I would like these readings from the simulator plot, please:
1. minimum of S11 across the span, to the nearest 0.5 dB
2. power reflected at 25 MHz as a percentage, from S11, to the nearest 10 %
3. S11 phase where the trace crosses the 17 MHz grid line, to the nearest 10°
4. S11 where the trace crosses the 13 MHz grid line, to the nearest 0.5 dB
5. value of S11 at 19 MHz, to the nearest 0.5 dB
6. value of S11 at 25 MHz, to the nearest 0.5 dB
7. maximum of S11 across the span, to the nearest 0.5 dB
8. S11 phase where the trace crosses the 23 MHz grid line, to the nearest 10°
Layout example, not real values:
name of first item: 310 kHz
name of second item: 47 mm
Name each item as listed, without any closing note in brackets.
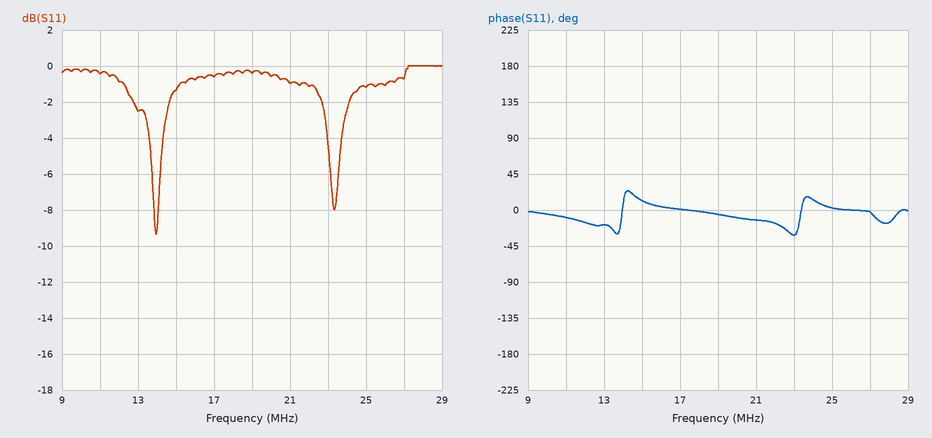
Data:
minimum of S11 across the span, to the nearest 0.5 dB: -9.5 dB
power reflected at 25 MHz as a percentage, from S11, to the nearest 10 %: 80 %
S11 phase where the trace crosses the 17 MHz grid line, to the nearest 10°: 0°
S11 where the trace crosses the 13 MHz grid line, to the nearest 0.5 dB: -2.5 dB
value of S11 at 19 MHz, to the nearest 0.5 dB: -0.5 dB
value of S11 at 25 MHz, to the nearest 0.5 dB: -1.0 dB
maximum of S11 across the span, to the nearest 0.5 dB: 0.0 dB
S11 phase where the trace crosses the 23 MHz grid line, to the nearest 10°: -30°
